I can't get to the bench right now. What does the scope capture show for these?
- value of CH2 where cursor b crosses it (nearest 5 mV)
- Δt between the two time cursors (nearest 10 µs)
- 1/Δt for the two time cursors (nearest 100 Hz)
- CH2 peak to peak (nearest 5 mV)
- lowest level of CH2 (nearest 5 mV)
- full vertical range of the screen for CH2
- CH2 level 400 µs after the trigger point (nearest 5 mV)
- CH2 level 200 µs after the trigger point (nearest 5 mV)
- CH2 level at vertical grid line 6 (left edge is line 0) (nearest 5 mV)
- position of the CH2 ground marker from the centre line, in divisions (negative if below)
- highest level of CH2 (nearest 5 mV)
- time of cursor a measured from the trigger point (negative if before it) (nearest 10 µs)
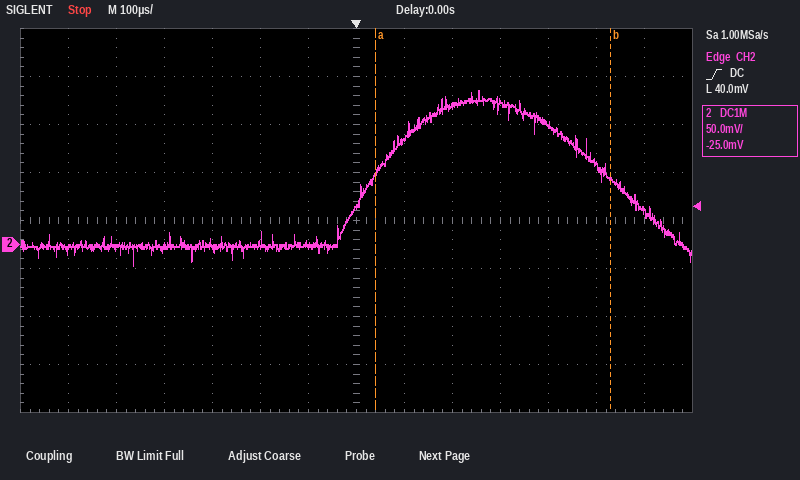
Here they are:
70 mV
490 µs
2.0 kHz
180 mV
-20 mV
400 mV
125 mV
145 mV
0 mV
-0.5 div
160 mV
+40 µs
